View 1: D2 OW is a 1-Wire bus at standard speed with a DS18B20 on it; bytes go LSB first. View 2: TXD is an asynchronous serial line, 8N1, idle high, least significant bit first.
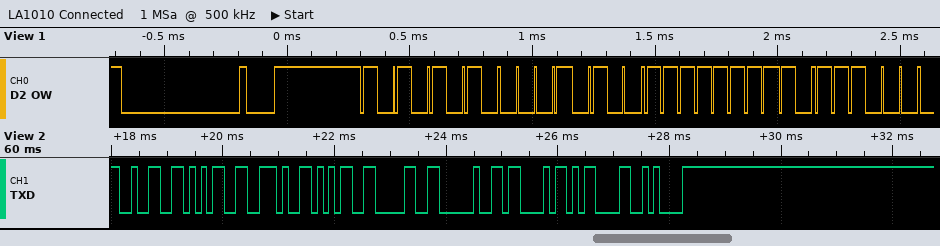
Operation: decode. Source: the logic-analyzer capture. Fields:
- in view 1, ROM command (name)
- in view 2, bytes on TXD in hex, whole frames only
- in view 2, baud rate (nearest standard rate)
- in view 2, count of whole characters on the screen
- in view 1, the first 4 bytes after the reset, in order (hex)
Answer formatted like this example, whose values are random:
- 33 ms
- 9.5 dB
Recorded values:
- Match ROM
- 0x32 0x35 0x2E 0x35 0x30 0x20 0x43 0x0D 0x0A
- 9600 baud
- 9
- 55 28 FF 1D
